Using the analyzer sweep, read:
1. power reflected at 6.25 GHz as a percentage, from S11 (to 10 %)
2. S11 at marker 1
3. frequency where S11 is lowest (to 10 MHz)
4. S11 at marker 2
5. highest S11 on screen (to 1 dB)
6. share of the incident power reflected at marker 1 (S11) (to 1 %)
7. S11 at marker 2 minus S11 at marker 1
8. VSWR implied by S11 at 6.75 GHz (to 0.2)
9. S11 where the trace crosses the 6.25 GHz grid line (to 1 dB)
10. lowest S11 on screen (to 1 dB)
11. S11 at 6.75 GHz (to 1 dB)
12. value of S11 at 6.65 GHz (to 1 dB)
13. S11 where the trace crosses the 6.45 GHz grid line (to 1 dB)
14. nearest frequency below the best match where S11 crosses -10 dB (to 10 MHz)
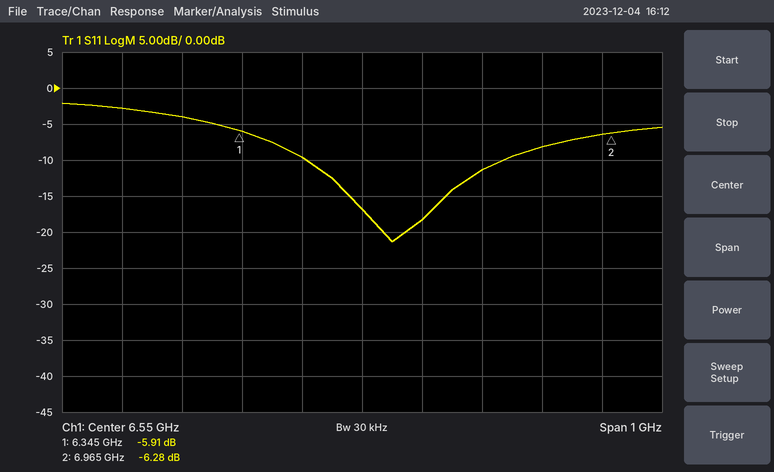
40 %
-5.91 dB
6.60 GHz
-6.28 dB
-2 dB
26 %
-0.37 dB
1.8
-4 dB
-21 dB
-11 dB
-18 dB
-10 dB
6.46 GHz
